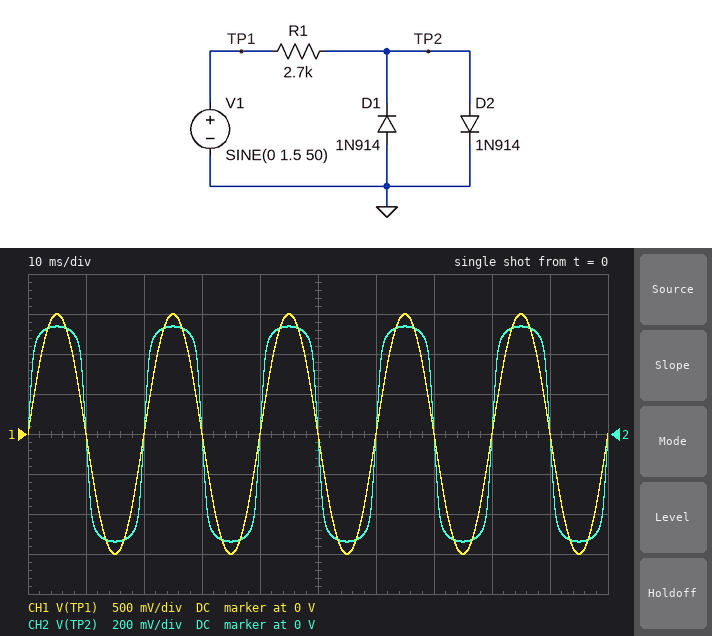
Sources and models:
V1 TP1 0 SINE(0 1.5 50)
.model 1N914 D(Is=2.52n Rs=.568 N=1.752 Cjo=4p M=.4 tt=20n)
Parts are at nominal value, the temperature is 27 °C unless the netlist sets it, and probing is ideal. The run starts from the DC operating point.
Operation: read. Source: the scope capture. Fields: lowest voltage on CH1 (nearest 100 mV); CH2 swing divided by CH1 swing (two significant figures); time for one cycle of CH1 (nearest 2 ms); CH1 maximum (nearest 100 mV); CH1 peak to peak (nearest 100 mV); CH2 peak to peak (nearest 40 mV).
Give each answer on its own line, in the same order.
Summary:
-1.5 V
0.36
20 ms
1.5 V
3.0 V
1.08 V
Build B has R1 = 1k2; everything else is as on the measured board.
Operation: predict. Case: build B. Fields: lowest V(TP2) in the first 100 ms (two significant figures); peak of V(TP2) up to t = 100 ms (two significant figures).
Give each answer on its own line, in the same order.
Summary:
-570 mV
570 mV
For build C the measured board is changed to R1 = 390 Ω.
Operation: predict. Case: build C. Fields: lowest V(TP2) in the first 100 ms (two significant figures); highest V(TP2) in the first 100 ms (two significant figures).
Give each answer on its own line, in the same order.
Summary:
-620 mV
620 mV
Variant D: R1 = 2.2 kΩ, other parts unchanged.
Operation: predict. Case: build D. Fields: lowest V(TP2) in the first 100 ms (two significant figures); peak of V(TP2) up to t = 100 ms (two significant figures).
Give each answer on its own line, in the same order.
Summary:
-550 mV
550 mV
